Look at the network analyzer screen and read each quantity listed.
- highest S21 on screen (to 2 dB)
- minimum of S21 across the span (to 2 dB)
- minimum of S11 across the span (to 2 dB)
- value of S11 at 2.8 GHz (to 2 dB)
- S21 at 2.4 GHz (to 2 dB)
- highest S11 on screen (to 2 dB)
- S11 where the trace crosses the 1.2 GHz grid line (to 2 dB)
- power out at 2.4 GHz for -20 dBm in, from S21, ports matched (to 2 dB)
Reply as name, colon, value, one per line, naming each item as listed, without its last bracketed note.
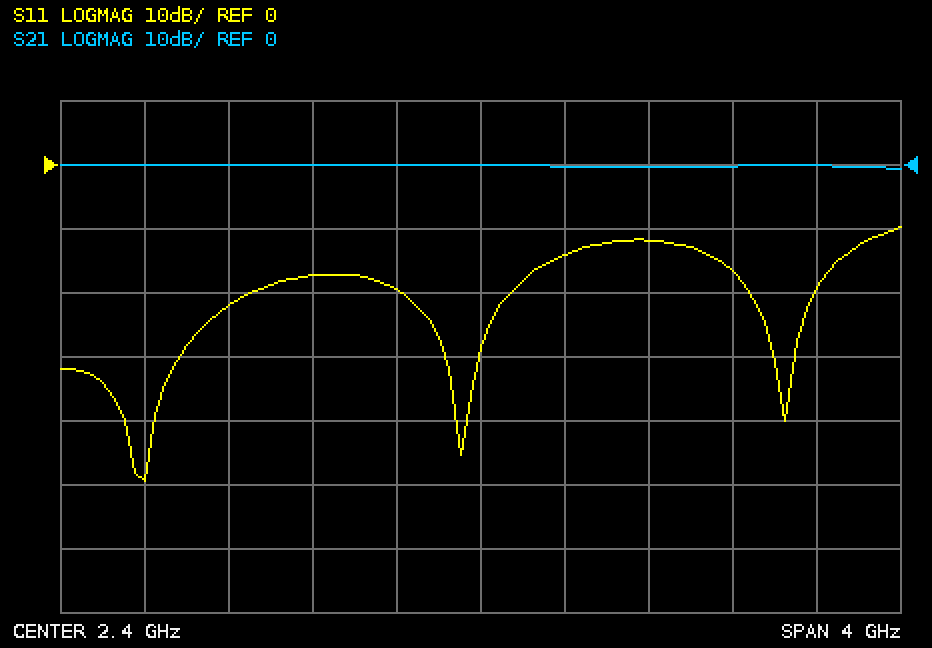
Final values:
highest S21 on screen: 0 dB
minimum of S21 across the span: 0 dB
minimum of S11 across the span: -50 dB
value of S11 at 2.8 GHz: -14 dB
S21 at 2.4 GHz: 0 dB
highest S11 on screen: -10 dB
S11 where the trace crosses the 1.2 GHz grid line: -22 dB
power out at 2.4 GHz for -20 dBm in, from S21, ports matched: -20 dBm
